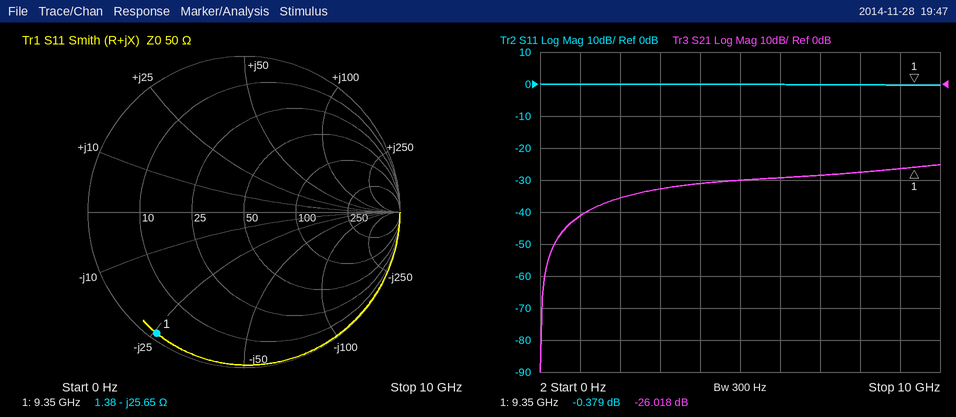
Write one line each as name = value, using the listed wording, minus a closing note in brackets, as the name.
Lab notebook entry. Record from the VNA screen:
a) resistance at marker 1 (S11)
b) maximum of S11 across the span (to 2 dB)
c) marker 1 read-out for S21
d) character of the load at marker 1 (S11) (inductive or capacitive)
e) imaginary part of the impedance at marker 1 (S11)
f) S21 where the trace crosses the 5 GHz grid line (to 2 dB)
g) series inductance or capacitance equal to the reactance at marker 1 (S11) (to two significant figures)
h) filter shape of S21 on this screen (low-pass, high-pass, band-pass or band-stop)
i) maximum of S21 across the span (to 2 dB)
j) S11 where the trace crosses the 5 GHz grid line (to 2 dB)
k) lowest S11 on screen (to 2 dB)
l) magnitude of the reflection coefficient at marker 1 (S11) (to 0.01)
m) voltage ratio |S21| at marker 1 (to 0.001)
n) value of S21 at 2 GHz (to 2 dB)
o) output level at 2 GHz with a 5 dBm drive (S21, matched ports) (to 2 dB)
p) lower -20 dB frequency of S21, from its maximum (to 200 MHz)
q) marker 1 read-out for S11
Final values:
resistance at marker 1 = 1.38 Ω
maximum of S11 across the span = 0 dB
marker 1 read-out for S21 = -26.018 dB
character of the load at marker 1 (S11) = capacitive
imaginary part of the impedance at marker 1 = -25.65 Ω
S21 where the trace crosses the 5 GHz grid line = -30 dB
series inductance or capacitance equal to the reactance at marker 1 (S11) = 660 fF
filter shape of S21 on this screen = high-pass
maximum of S21 across the span = -26 dB
S11 where the trace crosses the 5 GHz grid line = 0 dB
lowest S11 on screen = 0 dB
magnitude of the reflection coefficient at marker 1 (S11) = 0.96
voltage ratio |S21| at marker 1 = 0.050
value of S21 at 2 GHz = -36 dB
output level at 2 GHz with a 5 dBm drive (S21, matched ports) = -30 dBm
lower -20 dB frequency of S21, from its maximum = 600 MHz
marker 1 read-out for S11 = -0.379 dB
